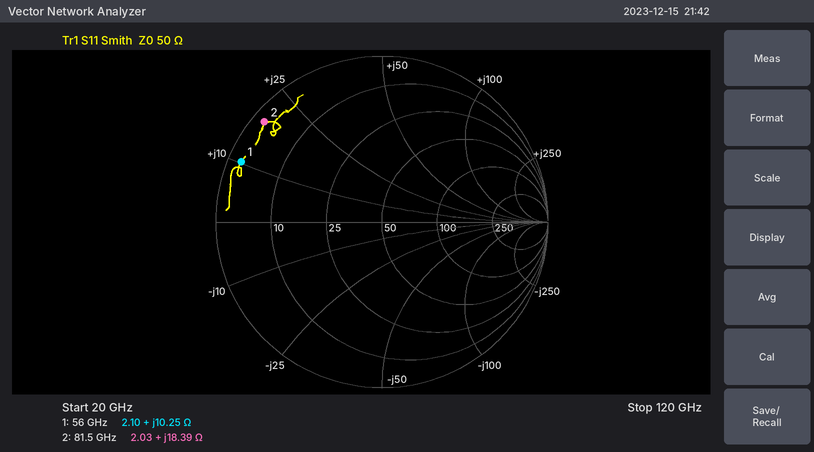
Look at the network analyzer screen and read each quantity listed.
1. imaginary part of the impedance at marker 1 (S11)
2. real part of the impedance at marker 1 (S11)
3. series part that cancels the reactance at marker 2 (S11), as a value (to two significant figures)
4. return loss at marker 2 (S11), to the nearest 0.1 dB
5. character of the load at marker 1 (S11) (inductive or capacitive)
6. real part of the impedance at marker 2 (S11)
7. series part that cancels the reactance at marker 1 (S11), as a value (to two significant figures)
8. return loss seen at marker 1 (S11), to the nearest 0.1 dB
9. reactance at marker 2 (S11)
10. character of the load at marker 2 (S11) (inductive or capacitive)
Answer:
+10.25 Ω
2.10 Ω
110 fF
0.6 dB
inductive
2.03 Ω
280 fF
0.7 dB
+18.39 Ω
inductive
